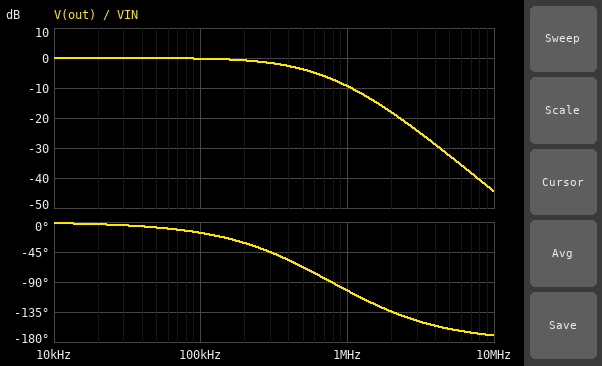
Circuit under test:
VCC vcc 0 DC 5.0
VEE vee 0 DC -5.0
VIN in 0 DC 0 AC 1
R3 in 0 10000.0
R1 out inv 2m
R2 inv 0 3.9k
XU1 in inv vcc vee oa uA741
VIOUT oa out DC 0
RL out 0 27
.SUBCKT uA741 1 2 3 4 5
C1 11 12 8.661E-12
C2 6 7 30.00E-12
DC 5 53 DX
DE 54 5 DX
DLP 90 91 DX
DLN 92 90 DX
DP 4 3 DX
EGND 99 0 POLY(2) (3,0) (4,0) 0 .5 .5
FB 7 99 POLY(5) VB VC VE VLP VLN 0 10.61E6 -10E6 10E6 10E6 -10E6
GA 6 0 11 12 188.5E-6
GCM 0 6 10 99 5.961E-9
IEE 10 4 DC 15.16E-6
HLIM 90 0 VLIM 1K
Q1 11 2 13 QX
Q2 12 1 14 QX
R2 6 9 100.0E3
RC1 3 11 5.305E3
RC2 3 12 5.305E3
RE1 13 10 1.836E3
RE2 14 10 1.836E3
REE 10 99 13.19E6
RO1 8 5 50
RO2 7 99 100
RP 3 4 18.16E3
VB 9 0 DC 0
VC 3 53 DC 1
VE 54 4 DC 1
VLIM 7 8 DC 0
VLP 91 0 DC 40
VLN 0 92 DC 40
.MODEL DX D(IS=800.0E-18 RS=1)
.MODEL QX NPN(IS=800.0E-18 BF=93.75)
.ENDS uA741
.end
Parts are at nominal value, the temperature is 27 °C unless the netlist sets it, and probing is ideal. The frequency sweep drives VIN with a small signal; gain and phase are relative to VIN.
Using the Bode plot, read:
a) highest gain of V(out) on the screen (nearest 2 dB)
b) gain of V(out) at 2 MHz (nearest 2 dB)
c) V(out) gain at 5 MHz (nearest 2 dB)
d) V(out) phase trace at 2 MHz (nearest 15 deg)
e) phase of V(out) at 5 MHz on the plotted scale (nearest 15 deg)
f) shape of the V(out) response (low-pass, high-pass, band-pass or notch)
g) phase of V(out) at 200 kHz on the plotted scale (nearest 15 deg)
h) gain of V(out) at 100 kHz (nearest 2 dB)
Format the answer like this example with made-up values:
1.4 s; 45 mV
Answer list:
0 dB; -18 dB; -32 dB; -135 deg; -165 deg; low-pass; -30 deg; 0 dB
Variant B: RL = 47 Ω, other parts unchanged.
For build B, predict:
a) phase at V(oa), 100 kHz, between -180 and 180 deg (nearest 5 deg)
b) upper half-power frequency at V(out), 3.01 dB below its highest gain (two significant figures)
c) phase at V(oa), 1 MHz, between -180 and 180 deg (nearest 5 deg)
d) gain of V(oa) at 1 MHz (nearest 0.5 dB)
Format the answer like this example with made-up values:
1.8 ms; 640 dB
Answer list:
-10 deg; 630 kHz; -95 deg; -6.5 dB
